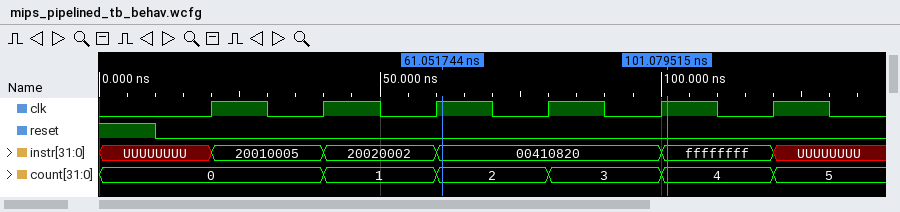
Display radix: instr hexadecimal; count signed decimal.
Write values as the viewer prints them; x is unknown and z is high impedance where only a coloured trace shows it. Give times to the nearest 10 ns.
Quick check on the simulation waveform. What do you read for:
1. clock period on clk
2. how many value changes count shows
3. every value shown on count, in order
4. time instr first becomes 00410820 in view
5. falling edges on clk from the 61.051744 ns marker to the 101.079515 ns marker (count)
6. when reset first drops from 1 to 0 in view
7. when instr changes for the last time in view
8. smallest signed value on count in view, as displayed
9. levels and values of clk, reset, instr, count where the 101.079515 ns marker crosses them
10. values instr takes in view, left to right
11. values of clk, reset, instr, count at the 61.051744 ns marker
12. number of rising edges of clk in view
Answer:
20 ns
5
0, 1, 2, 3, 4, 5
60 ns
2
10 ns
120 ns
0
clk=1, reset=0, instr=ffffffff, count=4
UUUUUUUU, 20010005, 20020002, 00410820, ffffffff, UUUUUUUU
clk=1, reset=0, instr=00410820, count=2
6
